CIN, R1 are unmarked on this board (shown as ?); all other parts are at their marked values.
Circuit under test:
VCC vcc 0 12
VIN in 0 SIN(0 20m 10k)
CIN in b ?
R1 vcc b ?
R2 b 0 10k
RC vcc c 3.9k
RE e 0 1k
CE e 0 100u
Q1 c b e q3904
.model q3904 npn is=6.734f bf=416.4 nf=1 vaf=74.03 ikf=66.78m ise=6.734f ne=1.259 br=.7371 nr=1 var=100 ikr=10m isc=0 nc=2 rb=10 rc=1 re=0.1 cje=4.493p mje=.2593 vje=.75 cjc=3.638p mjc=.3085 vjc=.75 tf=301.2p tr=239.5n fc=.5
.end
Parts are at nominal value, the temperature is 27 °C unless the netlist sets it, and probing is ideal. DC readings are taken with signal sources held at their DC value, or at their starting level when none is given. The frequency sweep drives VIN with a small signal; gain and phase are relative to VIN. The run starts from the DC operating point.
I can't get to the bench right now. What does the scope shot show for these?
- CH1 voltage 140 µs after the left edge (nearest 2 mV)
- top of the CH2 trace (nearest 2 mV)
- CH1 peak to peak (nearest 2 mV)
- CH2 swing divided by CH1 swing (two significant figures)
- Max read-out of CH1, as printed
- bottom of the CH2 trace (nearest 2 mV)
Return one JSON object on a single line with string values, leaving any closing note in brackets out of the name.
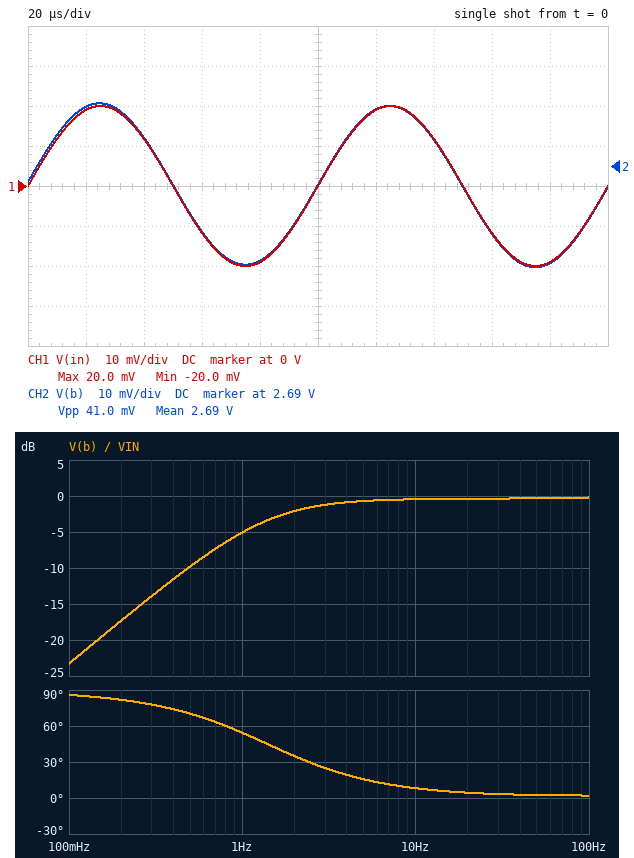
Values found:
{"CH1 voltage 140 µs after the left edge": "12 mV", "top of the CH2 trace": "2.706 V", "CH1 peak to peak": "40 mV", "CH2 swing divided by CH1 swing": "1.0", "Max read-out of CH1, as printed": "20.0 mV", "bottom of the CH2 trace": "2.664 V"}
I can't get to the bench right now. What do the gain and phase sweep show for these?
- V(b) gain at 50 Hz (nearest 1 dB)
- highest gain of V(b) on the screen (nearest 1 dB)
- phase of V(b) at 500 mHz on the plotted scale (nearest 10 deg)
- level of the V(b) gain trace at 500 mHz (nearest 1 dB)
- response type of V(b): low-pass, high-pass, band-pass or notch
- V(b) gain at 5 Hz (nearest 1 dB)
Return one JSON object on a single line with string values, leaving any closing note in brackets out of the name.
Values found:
{"V(b) gain at 50 Hz": "0 dB", "highest gain of V(b) on the screen": "0 dB", "phase of V(b) at 500 mHz on the plotted scale": "70 deg", "level of the V(b) gain trace at 500 mHz": "-10 dB", "response type of V(b): low-pass, high-pass, band-pass or notch": "high-pass", "V(b) gain at 5 Hz": "-1 dB"}
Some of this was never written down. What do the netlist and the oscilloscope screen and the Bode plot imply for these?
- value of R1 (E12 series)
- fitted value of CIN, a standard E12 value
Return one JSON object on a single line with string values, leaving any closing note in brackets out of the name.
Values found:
{"value of R1": "33 kΩ", "fitted value of CIN, a standard E12 value": "15 µF"}
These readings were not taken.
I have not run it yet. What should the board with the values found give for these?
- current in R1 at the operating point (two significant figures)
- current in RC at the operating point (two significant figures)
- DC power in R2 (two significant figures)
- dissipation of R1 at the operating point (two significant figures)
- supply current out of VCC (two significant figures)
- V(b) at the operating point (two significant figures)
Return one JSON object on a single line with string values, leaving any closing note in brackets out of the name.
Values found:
{"current in R1 at the operating point": "280 µA", "current in RC at the operating point": "2.0 mA", "DC power in R2": "720 µW", "dissipation of R1 at the operating point": "2.6 mW", "supply current out of VCC": "2.3 mA", "V(b) at the operating point": "2.7 V"}
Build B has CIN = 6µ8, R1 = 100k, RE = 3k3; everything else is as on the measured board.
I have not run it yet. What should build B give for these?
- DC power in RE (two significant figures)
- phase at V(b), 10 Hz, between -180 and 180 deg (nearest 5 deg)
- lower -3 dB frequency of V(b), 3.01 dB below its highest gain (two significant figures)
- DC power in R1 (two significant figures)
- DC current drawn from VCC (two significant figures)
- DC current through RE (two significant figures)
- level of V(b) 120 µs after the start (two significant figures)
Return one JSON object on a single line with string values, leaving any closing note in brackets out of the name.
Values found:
{"DC power in RE": "66 µW", "phase at V(b), 10 Hz, between -180 and 180 deg": "15 deg", "lower -3 dB frequency of V(b), 3.01 dB below its highest gain": "3.0 Hz", "DC power in R1": "1.2 mW", "DC current drawn from VCC": "250 µA", "DC current through RE": "140 µA", "level of V(b) 120 µs after the start": "1.1 V"}
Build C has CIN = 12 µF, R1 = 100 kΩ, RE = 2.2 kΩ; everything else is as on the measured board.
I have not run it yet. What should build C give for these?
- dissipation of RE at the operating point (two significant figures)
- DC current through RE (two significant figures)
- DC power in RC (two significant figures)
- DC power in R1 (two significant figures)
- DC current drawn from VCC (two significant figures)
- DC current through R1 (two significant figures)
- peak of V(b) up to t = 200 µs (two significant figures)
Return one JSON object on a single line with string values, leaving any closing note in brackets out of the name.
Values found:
{"dissipation of RE at the operating point": "94 µW", "DC current through RE": "210 µA", "DC power in RC": "160 µW", "DC power in R1": "1.2 mW", "DC current drawn from VCC": "310 µA", "DC current through R1": "110 µA", "peak of V(b) up to t = 200 µs": "1.1 V"}
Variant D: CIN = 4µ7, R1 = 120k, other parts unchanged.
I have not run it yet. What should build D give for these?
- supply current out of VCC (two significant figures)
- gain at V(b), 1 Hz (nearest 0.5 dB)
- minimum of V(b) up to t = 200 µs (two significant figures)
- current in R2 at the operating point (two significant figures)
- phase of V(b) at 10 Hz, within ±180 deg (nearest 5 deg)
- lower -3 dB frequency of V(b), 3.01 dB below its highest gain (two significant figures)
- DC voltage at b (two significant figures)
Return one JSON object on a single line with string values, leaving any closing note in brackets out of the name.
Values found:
{"supply current out of VCC": "360 µA", "gain at V(b), 1 Hz": "-12.0 dB", "minimum of V(b) up to t = 200 µs": "880 mV", "current in R2 at the operating point": "90 µA", "phase of V(b) at 10 Hz, within ±180 deg": "20 deg", "lower -3 dB frequency of V(b), 3.01 dB below its highest gain": "4.6 Hz", "DC voltage at b": "900 mV"}
